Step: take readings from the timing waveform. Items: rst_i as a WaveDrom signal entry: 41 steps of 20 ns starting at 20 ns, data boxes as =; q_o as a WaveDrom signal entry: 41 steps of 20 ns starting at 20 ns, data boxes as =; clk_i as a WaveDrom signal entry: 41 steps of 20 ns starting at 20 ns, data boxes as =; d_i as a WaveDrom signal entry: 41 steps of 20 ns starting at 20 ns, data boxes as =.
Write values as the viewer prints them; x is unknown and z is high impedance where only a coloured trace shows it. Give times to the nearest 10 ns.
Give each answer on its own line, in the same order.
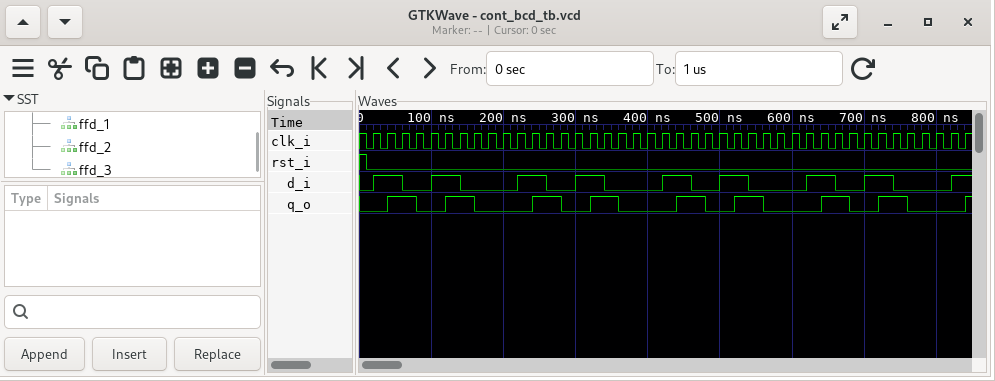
{name: 'rst_i', wave: '0........................................'}
{name: 'q_o', wave: '01.0.1.0...1.0.1.0...1.0.1.0...1.0.1.0...'}
{name: 'clk_i', wave: 'p........................................'}
{name: 'd_i', wave: '1.0.1.0...1.0.1.0...1.0.1.0...1.0.1.0...1'}
